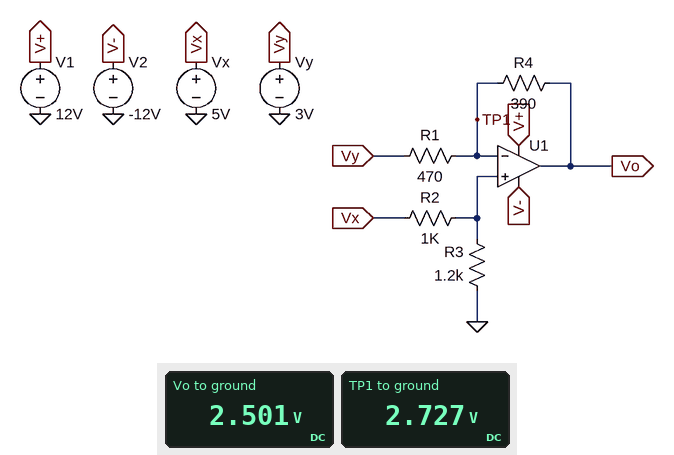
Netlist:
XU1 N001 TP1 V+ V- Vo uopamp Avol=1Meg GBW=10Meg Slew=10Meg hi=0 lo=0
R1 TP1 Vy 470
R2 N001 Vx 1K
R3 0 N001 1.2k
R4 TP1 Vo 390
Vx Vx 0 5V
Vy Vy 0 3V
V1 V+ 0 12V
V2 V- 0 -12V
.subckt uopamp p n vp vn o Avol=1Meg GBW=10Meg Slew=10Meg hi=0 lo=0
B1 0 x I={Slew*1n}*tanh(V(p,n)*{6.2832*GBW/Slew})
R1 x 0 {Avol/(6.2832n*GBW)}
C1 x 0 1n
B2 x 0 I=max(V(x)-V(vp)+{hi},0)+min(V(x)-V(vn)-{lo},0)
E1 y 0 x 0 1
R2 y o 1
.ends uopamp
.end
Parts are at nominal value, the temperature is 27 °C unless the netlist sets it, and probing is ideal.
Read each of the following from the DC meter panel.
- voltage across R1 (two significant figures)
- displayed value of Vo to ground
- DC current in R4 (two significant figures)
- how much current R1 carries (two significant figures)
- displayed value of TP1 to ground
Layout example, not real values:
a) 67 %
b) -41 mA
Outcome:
a) 270 mV
b) 2.501 V
c) 580 µA
d) 580 µA
e) 2.727 V
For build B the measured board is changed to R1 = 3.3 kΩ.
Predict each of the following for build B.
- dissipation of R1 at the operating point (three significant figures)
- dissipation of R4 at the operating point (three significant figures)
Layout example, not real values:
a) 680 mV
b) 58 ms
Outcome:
a) 22.5 µW
b) 2.66 µW
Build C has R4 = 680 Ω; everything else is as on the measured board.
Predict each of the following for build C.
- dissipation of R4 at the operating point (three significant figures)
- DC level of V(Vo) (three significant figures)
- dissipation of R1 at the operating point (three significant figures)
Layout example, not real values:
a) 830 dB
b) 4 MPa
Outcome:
a) 229 µW
b) 2.33 V
c) 158 µW
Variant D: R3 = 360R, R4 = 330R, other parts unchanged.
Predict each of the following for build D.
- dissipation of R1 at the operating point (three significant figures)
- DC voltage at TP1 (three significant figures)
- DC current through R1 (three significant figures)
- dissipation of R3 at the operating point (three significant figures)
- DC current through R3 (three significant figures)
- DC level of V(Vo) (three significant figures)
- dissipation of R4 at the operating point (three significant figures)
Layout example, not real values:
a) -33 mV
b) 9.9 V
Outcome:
a) 5.98 mW
b) 1.32 V
c) 3.57 mA
d) 4.87 mW
e) 3.68 mA
f) 146 mV
g) 4.20 mW
